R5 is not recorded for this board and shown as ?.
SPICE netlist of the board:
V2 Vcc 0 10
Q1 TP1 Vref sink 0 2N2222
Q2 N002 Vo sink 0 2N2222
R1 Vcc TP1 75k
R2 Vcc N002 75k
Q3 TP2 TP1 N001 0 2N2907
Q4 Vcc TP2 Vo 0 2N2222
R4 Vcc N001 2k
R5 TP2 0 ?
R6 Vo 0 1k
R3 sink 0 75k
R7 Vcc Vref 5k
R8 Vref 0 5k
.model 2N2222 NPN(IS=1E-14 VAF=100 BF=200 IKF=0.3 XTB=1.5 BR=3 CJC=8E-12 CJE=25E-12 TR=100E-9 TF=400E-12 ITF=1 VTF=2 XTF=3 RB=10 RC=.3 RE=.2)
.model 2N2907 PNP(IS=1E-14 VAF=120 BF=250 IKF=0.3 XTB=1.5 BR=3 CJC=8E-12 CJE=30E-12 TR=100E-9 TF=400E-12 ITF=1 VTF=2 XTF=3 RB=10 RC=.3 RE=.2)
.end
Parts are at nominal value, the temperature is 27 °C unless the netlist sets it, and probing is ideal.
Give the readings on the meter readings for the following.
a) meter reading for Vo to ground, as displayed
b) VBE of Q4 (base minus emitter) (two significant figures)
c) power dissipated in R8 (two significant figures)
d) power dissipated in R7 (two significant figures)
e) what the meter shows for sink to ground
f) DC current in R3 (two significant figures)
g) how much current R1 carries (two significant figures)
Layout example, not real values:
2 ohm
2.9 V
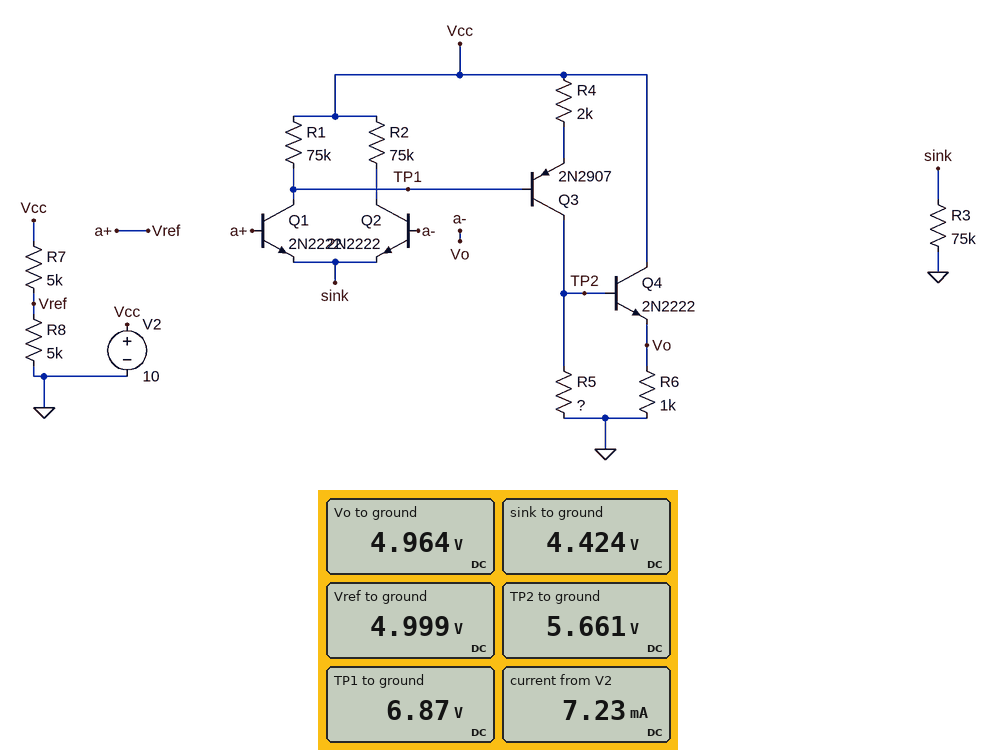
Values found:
4.964 V
700 mV
5.0 mW
5.0 mW
4.424 V
59 µA
42 µA
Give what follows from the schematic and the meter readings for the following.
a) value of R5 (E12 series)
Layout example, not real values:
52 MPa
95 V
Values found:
4.7 kΩ
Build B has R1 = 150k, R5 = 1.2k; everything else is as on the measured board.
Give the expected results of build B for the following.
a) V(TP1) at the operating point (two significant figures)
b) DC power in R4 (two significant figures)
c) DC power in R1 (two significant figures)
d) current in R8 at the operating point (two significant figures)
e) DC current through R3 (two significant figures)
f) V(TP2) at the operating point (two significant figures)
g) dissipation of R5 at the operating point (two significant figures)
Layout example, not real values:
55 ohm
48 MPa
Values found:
4.4 V
12 mW
210 µW
990 µA
58 µA
2.9 V
7.1 mW
